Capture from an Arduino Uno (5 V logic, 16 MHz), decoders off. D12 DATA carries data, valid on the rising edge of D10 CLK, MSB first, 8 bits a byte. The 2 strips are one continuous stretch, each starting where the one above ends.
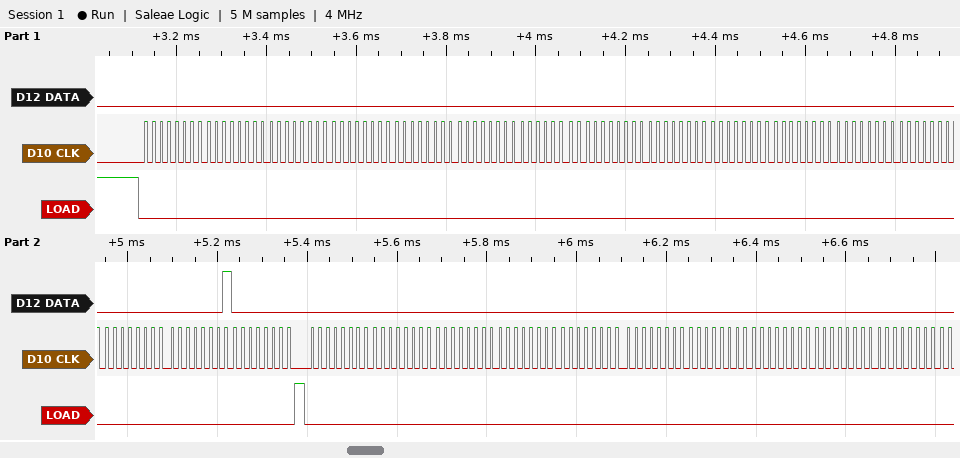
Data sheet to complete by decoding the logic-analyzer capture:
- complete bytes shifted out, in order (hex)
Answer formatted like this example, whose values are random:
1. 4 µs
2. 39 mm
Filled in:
1. 0x00 0x00 0x00 0x00 0x00 0x00 0x00 0x00 0x00 0x00 0x00 0x00 0x00 0x00 0x01 0x00 0x00 0x00 0x00 0x00 0x00 0x00 0x00 0x00 0x00 0x00
